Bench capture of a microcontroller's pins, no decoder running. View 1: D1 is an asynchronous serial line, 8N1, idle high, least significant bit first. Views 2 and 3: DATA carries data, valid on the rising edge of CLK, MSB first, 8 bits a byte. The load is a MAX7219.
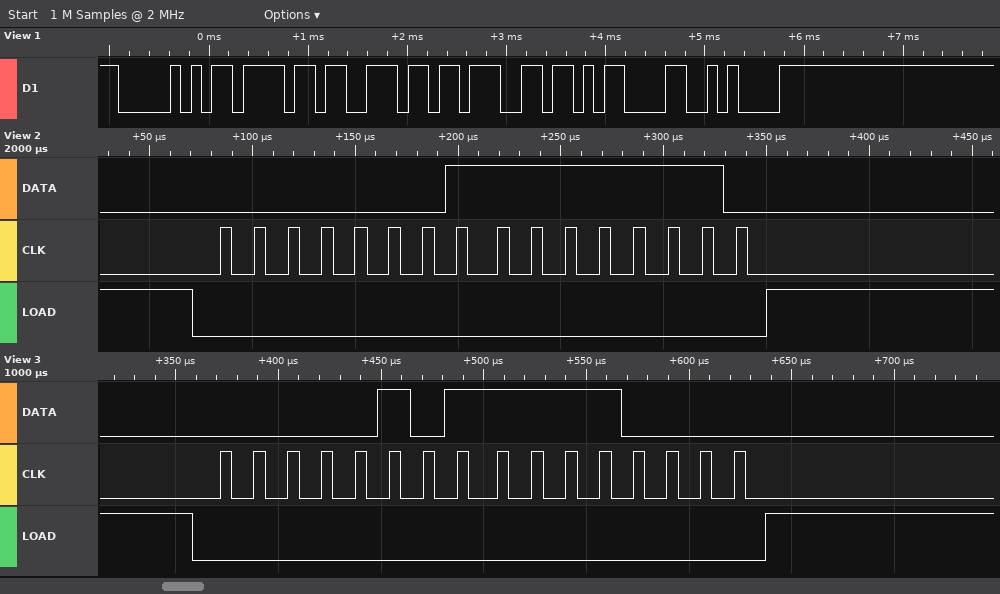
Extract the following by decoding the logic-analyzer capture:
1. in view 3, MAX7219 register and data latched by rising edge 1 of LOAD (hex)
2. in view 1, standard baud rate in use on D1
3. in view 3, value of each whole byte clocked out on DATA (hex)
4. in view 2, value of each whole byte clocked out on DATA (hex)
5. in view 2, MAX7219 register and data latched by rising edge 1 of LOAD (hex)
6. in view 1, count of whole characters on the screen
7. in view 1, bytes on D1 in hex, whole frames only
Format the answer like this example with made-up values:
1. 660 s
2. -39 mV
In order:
1. register 0x5, data 0xF0
2. 9600 baud
3. 05 F0
4. 01 FE
5. register 0x1, data 0xFE
6. 6
7. 0x50 0x6F 0x6E 0x67 0x0D 0x0A
